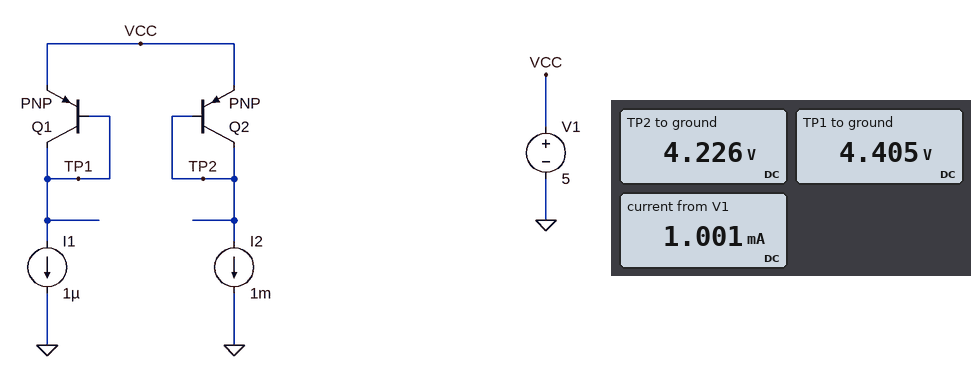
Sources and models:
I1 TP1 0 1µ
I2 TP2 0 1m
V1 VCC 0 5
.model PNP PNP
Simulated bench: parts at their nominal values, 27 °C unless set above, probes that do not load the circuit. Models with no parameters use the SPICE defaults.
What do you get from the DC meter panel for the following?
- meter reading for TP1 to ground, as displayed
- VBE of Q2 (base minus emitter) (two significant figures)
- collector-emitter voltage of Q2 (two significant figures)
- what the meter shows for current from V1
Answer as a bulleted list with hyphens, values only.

- 4.405 V
- -770 mV
- -770 mV
- 1.001 mA
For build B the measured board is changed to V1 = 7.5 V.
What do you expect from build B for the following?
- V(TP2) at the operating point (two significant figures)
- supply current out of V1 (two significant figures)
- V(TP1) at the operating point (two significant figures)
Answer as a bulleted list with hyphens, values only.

- 6.7 V
- 1.0 mA
- 6.9 V
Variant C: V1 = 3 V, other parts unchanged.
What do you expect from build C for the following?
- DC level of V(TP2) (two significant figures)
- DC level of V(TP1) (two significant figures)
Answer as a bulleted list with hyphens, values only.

- 2.2 V
- 2.4 V
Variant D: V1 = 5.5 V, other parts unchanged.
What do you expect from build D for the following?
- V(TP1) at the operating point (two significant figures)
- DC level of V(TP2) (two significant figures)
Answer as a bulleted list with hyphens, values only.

- 4.9 V
- 4.7 V
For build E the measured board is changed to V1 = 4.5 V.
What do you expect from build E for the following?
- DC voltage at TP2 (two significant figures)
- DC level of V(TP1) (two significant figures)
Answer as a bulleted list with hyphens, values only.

- 3.7 V
- 3.9 V
